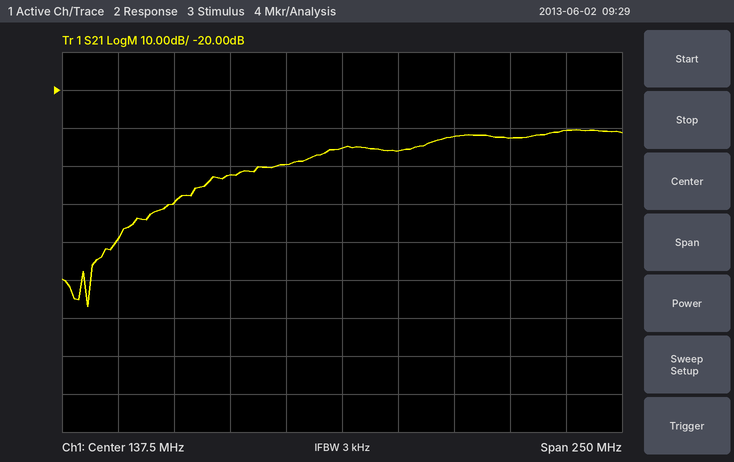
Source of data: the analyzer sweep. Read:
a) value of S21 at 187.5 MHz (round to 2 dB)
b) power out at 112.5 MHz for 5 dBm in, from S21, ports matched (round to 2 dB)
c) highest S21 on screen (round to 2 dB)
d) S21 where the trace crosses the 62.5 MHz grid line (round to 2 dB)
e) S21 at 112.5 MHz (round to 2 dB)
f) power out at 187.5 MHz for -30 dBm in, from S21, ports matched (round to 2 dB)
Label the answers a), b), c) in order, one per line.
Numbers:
a) -32 dB
b) -34 dBm
c) -30 dB
d) -50 dB
e) -40 dB
f) -62 dBm
